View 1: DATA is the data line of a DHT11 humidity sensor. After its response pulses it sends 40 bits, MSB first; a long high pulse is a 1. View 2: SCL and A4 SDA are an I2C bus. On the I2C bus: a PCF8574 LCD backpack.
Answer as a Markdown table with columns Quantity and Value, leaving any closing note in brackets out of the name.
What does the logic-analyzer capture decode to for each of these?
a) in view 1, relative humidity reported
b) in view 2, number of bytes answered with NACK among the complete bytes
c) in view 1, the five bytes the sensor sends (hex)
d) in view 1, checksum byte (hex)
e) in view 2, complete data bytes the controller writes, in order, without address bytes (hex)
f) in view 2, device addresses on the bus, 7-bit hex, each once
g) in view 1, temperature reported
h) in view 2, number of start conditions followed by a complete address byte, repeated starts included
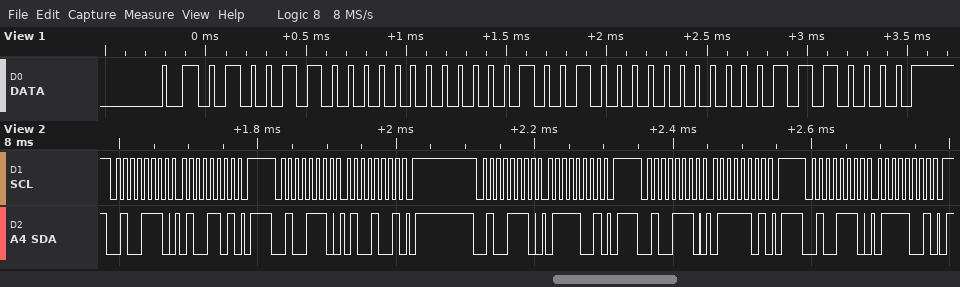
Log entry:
| Quantity | Value |
|---|---|
| in view 1, relative humidity reported | 76 % |
| in view 2, number of bytes answered with NACK among the complete bytes | 0 |
| in view 1, the five bytes the sensor sends | 4C 00 24 00 70 |
| in view 1, checksum byte | 0x70 |
| in view 2, complete data bytes the controller writes, in order, without address bytes | 4D 49 79 7D 79 |
| in view 2, device addresses on the bus, 7-bit hex, each once | 0x27 |
| in view 1, temperature reported | 36.0 °C |
| in view 2, number of start conditions followed by a complete address byte, repeated starts included | 5 |
